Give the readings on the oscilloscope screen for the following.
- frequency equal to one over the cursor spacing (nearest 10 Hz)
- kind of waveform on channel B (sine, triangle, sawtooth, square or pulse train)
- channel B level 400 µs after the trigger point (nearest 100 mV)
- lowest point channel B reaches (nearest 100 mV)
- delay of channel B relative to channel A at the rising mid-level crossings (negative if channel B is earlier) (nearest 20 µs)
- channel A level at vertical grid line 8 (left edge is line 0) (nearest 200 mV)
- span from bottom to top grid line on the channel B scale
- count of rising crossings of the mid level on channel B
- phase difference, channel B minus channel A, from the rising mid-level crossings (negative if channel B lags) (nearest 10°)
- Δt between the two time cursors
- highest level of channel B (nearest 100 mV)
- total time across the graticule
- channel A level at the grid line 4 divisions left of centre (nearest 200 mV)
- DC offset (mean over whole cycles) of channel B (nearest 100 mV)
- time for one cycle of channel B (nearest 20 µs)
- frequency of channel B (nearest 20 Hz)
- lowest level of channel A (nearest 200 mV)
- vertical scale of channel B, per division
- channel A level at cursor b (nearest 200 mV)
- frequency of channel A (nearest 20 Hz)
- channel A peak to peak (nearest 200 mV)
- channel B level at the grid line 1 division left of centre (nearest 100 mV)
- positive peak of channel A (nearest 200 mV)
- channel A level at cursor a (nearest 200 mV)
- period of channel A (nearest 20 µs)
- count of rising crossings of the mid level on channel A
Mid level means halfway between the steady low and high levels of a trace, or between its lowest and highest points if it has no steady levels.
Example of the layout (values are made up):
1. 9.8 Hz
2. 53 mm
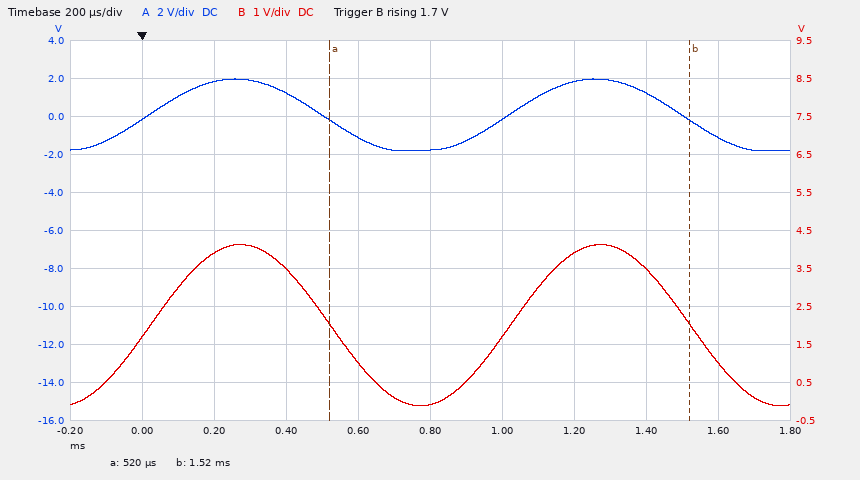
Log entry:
1. 1.00 kHz
2. sine
3. 3.5 V
4. -100 mV
5. 0 µs
6. 1.2 V
7. 10 V
8. 2
9. 0°
10. 1.00 ms
11. 4.1 V
12. 2 ms
13. -200 mV
14. 2.0 V
15. 1.00 ms
16. 1.00 kHz
17. -1.8 V
18. 1 V
19. -200 mV
20. 1.00 kHz
21. 3.8 V
22. 1.0 V
23. 2.0 V
24. -200 mV
25. 1.00 ms
26. 2
